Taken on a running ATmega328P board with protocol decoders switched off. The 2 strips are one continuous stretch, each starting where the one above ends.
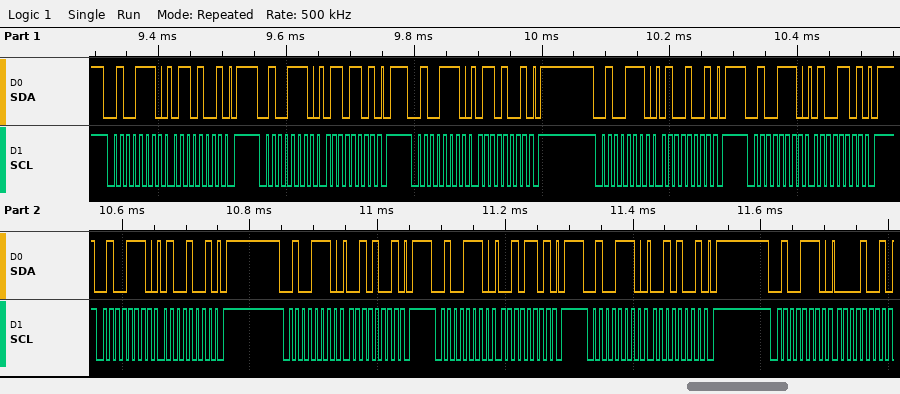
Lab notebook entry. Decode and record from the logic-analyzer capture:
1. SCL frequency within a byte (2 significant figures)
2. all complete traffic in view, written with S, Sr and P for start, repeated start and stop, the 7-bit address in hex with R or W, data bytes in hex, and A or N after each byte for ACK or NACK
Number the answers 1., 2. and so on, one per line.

1. 100 kHz
2. S 27W A 69 A P S 27W A 6D A P S 27W A 69 A P S 27W A 49 A P S 27W A 4D A P S 27W A 49 A P S 27W A 29 A P S 27W A 2D A P S 27W A 29 A P S 27W A 09 A
